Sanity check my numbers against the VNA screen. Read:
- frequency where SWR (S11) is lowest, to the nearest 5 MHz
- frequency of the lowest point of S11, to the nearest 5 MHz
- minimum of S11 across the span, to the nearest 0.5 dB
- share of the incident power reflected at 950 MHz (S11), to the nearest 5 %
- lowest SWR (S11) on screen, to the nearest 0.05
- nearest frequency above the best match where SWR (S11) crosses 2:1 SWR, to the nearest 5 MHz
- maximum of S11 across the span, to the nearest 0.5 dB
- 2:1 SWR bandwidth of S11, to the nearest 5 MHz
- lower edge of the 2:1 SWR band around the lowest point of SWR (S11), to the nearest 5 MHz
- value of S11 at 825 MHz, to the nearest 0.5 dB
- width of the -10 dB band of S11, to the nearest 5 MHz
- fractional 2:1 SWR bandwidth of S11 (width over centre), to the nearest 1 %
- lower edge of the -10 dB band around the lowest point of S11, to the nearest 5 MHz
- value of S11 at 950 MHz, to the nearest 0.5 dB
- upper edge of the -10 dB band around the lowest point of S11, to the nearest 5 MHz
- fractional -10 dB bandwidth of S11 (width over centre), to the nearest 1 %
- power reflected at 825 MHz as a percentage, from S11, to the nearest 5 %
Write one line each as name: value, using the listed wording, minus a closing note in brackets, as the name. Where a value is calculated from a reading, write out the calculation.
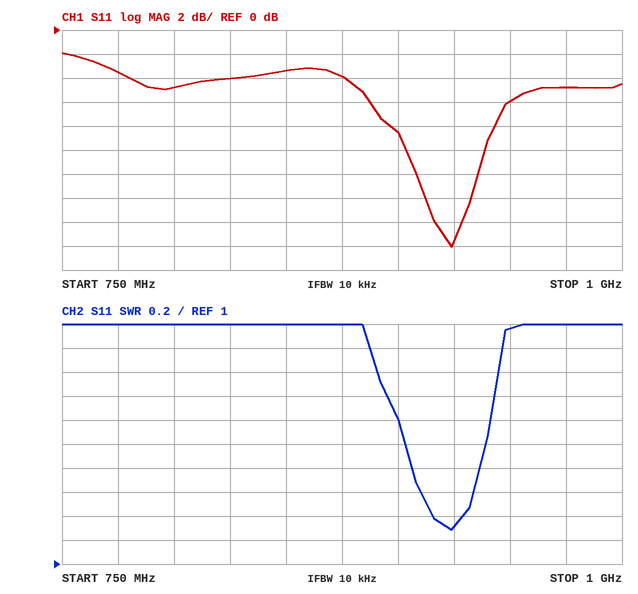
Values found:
frequency where SWR (S11) is lowest, to the nearest 5 MHz: 925 MHz
frequency of the lowest point of S11, to the nearest 5 MHz: 925 MHz
minimum of S11 across the span, to the nearest 0.5 dB: -18.0 dB
share of the incident power reflected at 950 MHz (S11), to the nearest 5 %: 10^(-6/10) ≈ 25 %
lowest SWR (S11) on screen, to the nearest 0.05: 1.30
nearest frequency above the best match where SWR (S11) crosses 2:1 SWR, to the nearest 5 MHz: 940 MHz
maximum of S11 across the span, to the nearest 0.5 dB: -2.0 dB
2:1 SWR bandwidth of S11, to the nearest 5 MHz: 940 MHz − 905 MHz = 35 MHz
lower edge of the 2:1 SWR band around the lowest point of SWR (S11), to the nearest 5 MHz: 905 MHz
value of S11 at 825 MHz, to the nearest 0.5 dB: -4.0 dB
width of the -10 dB band of S11, to the nearest 5 MHz: 940 MHz − 905 MHz = 35 MHz
fractional 2:1 SWR bandwidth of S11 (width over centre), to the nearest 1 %: 35 MHz / 922.5 MHz ≈ 4 %
lower edge of the -10 dB band around the lowest point of S11, to the nearest 5 MHz: 905 MHz
value of S11 at 950 MHz, to the nearest 0.5 dB: -6.0 dB
upper edge of the -10 dB band around the lowest point of S11, to the nearest 5 MHz: 940 MHz
fractional -10 dB bandwidth of S11 (width over centre), to the nearest 1 %: 35 MHz / 922.5 MHz ≈ 4 %
power reflected at 825 MHz as a percentage, from S11, to the nearest 5 %: 10^(-4/10) ≈ 40 %
